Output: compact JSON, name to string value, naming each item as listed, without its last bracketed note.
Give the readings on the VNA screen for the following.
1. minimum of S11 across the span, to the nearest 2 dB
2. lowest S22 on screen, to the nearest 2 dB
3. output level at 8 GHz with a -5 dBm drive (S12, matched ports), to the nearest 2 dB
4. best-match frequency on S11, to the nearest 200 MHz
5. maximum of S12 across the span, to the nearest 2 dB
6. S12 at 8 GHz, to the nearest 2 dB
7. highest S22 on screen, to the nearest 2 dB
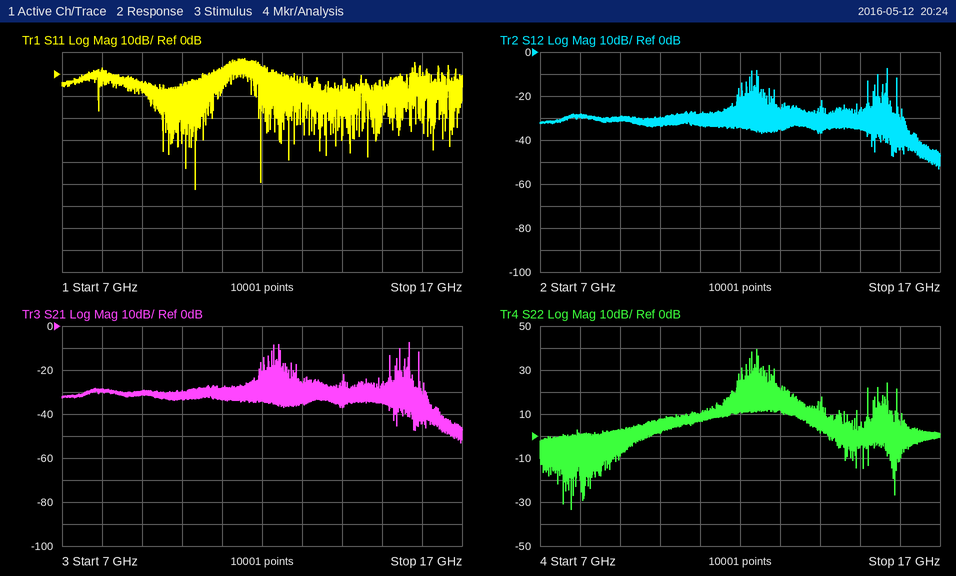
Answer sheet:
{"minimum of S11 across the span, to the nearest 2 dB": "-52 dB", "lowest S22 on screen, to the nearest 2 dB": "-34 dB", "output level at 8 GHz with a -5 dBm drive (S12, matched ports), to the nearest 2 dB": "-34 dBm", "best-match frequency on S11, to the nearest 200 MHz": "10.4 GHz", "maximum of S12 across the span, to the nearest 2 dB": "-8 dB", "S12 at 8 GHz, to the nearest 2 dB": "-28 dB", "highest S22 on screen, to the nearest 2 dB": "40 dB"}
